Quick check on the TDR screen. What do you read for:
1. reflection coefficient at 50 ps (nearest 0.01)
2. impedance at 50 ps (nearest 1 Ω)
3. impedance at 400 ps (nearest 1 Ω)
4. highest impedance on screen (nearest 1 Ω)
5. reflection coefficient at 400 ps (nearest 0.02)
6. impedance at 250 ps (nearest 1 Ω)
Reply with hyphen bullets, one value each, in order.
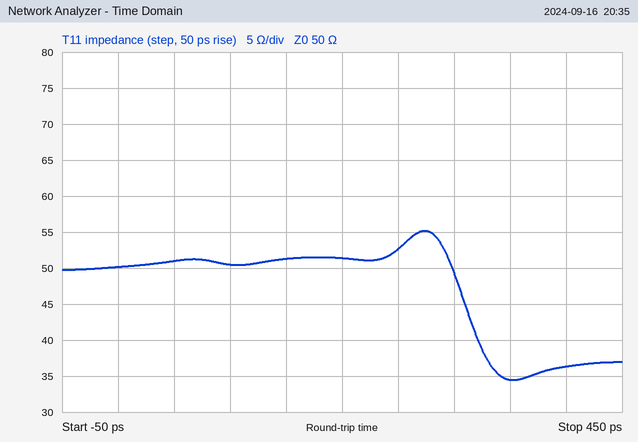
- +0.01
- 51 Ω
- 36 Ω
- 55 Ω
- -0.16
- 53 Ω
